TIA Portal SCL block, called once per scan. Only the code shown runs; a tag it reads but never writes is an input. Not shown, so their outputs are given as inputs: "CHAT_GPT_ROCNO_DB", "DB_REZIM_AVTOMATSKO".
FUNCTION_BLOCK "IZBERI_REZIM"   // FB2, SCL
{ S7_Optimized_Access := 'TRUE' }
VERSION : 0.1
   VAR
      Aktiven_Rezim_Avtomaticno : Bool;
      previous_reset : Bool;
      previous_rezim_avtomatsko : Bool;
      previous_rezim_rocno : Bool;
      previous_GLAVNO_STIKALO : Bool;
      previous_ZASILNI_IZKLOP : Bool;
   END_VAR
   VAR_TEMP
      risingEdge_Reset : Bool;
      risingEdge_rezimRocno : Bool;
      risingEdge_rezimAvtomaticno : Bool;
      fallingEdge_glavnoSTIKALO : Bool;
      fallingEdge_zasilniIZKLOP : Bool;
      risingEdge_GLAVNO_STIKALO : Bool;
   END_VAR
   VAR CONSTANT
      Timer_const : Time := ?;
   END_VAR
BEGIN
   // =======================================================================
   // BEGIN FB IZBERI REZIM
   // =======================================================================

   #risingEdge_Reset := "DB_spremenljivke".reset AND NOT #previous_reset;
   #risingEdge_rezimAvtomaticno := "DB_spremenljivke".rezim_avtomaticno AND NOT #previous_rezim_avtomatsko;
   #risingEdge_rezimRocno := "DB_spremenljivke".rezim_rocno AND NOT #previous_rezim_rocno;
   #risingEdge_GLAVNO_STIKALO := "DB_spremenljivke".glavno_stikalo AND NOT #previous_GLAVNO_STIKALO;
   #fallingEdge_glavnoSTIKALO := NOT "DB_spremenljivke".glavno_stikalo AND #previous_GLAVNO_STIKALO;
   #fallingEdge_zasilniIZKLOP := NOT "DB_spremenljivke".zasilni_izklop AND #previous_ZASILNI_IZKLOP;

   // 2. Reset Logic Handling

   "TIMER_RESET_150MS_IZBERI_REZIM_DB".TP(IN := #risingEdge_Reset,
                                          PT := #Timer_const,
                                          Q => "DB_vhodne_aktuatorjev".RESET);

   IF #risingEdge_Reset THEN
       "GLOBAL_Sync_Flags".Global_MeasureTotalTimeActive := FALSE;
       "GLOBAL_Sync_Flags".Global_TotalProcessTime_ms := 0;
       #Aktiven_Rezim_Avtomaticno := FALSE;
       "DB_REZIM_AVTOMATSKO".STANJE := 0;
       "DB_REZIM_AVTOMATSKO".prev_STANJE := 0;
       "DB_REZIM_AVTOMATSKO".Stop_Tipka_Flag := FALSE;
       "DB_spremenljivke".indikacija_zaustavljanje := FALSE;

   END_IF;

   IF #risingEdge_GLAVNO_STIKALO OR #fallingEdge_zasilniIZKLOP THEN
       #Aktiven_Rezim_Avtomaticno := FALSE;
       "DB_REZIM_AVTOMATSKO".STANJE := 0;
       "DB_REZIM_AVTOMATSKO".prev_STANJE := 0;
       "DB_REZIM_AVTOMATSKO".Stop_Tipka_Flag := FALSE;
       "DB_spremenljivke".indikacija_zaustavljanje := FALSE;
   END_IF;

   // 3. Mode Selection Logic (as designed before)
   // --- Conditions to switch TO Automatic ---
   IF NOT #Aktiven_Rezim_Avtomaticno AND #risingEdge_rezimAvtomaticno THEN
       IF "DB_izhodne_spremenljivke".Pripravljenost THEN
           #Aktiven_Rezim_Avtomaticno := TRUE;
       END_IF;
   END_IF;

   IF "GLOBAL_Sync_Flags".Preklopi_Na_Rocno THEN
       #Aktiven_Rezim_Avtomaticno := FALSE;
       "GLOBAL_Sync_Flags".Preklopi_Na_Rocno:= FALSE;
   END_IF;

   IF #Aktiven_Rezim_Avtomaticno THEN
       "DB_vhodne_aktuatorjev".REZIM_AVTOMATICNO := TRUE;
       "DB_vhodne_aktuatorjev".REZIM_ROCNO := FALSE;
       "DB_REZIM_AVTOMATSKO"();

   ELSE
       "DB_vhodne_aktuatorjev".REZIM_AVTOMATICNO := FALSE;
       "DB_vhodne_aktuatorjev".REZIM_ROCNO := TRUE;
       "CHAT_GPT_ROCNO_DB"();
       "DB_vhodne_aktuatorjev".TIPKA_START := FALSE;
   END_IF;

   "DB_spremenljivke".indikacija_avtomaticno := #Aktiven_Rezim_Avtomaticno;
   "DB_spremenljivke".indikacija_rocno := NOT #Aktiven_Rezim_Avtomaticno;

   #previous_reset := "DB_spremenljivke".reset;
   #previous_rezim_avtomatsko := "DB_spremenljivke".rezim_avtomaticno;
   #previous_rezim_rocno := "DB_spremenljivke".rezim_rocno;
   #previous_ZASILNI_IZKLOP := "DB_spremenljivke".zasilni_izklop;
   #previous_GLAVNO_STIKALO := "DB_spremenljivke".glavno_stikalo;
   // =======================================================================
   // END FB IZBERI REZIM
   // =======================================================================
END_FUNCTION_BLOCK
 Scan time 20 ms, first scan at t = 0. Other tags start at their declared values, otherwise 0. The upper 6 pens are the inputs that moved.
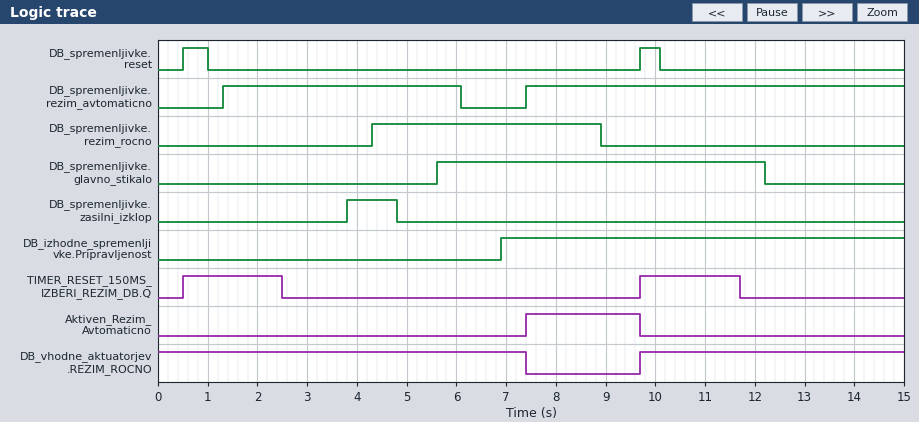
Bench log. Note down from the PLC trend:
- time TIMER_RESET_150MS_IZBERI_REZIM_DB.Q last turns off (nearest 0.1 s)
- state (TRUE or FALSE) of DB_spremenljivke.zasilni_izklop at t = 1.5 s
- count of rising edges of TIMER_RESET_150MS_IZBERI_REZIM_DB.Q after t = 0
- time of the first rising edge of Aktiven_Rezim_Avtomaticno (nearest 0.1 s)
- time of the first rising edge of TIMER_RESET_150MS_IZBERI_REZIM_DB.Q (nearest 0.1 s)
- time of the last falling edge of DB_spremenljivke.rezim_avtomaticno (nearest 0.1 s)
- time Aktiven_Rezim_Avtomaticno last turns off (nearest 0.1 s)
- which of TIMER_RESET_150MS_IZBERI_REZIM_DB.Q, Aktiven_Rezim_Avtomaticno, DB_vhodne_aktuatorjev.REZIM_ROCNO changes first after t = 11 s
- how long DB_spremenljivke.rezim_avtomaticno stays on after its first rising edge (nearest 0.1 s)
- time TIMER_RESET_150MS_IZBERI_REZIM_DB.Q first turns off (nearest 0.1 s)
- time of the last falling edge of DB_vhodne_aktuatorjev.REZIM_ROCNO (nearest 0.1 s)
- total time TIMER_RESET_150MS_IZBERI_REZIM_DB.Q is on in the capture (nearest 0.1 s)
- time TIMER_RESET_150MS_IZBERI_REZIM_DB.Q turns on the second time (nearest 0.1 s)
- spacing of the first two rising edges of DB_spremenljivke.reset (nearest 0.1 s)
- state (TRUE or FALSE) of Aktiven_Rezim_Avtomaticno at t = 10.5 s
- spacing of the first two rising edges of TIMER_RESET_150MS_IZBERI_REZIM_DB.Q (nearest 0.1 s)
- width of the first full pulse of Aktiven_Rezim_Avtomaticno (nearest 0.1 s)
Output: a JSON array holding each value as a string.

["11.7 s", "FALSE", "2", "7.4 s", "0.5 s", "6.1 s", "9.7 s", "TIMER_RESET_150MS_IZBERI_REZIM_DB.Q", "4.8 s", "2.5 s", "7.4 s", "4.0 s", "9.7 s", "9.2 s", "FALSE", "9.2 s", "2.3 s"]
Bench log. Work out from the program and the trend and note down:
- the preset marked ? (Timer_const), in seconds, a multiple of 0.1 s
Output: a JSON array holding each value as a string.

["2.0 s"]
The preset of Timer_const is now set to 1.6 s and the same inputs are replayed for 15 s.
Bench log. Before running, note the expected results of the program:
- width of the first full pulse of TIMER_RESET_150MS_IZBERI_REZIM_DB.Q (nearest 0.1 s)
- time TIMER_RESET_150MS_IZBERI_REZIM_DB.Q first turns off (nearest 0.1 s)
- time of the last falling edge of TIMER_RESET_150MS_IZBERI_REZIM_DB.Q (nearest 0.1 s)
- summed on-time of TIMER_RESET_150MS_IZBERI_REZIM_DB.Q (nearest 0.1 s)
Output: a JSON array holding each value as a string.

["1.6 s", "2.1 s", "11.3 s", "3.2 s"]
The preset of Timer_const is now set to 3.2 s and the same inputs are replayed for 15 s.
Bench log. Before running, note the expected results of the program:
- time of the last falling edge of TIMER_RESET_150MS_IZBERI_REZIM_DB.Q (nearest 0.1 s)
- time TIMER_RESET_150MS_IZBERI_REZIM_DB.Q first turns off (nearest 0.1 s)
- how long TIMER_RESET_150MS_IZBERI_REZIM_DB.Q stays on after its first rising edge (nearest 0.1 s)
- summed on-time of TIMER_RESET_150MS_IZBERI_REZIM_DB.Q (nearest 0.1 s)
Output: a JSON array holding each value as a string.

["12.9 s", "3.7 s", "3.2 s", "6.4 s"]
